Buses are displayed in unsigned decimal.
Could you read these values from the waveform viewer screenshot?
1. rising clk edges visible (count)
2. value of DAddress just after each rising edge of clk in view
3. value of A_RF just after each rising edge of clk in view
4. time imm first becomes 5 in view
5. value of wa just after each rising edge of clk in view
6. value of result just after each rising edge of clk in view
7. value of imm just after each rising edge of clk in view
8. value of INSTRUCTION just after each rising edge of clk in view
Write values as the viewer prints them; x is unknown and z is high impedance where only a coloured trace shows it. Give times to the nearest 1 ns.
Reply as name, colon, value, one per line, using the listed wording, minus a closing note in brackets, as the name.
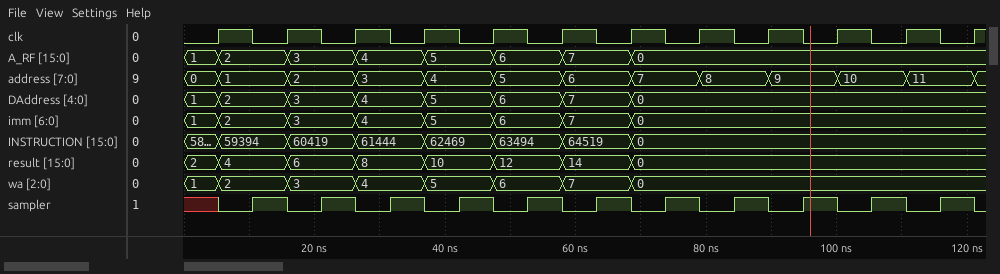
rising clk edges visible: 12
value of DAddress just after each rising edge of clk in view: 2, 3, 4, 5, 6, 7, 0, 0, 0, 0, 0, 0
value of A_RF just after each rising edge of clk in view: 2, 3, 4, 5, 6, 7, 0, 0, 0, 0, 0, 0
time imm first becomes 5 in view: 37 ns
value of wa just after each rising edge of clk in view: 2, 3, 4, 5, 6, 7, 0, 0, 0, 0, 0, 0
value of result just after each rising edge of clk in view: 4, 6, 8, 10, 12, 14, 0, 0, 0, 0, 0, 0
value of imm just after each rising edge of clk in view: 2, 3, 4, 5, 6, 7, 0, 0, 0, 0, 0, 0
value of INSTRUCTION just after each rising edge of clk in view: 59394, 60419, 61444, 62469, 63494, 64519, 0, 0, 0, 0, 0, 0
